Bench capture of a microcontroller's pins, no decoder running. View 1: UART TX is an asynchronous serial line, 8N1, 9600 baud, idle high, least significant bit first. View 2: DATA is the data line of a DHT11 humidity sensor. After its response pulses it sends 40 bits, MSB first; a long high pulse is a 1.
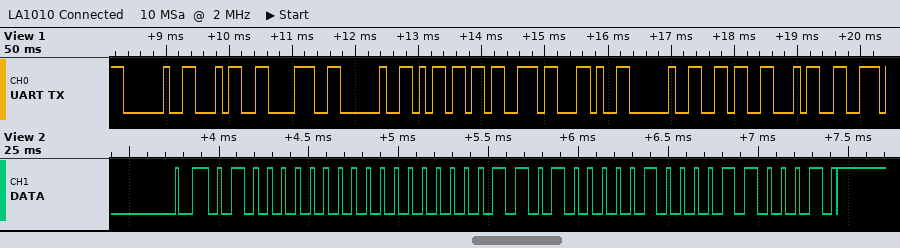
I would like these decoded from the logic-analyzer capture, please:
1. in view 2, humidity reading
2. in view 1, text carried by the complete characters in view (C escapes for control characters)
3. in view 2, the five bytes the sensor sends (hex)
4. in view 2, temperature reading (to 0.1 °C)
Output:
64 %
" 48 ms, 64"
40 00 1A 08 62
26.8 °C
